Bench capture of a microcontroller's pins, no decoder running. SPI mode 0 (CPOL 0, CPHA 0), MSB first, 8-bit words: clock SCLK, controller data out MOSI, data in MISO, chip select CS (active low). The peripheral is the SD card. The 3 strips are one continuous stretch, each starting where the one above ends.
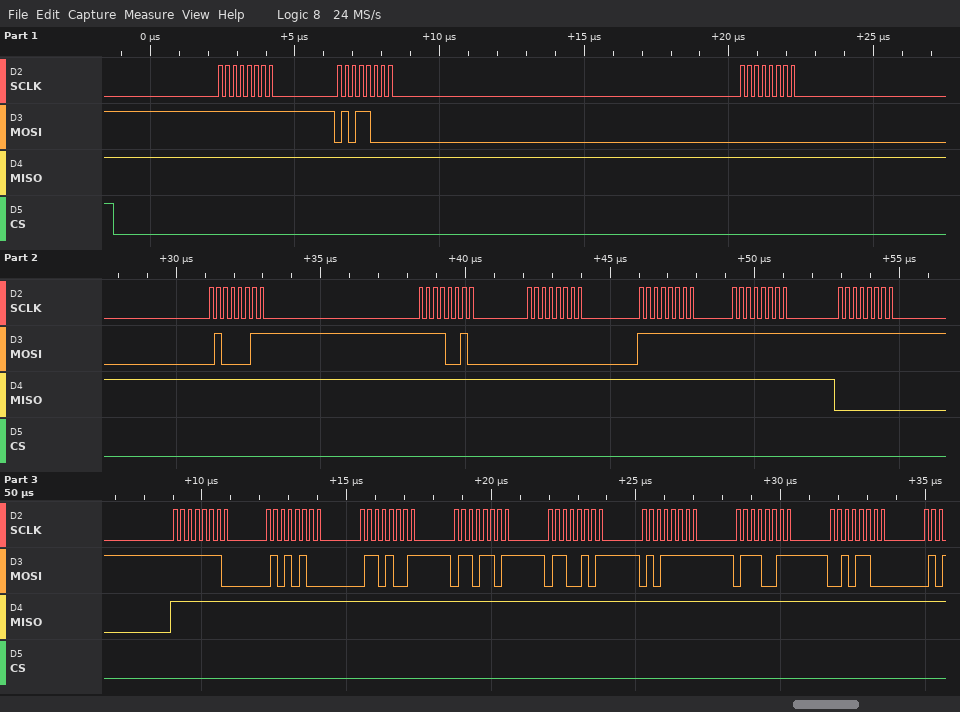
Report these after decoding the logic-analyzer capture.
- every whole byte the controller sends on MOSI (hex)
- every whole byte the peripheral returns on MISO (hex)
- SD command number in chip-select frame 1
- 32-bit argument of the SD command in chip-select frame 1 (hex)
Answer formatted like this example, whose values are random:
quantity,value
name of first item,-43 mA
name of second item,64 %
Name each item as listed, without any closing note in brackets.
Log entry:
quantity,value
every whole byte the controller sends on MOSI,0xFF 0x58 0x00 0x43 0xF2 0x00 0xFF 0xFF 0xFF 0xFE 0x54 0x69 0x6D 0x65 0x5F 0x73 0x2C
every whole byte the peripheral returns on MISO,0xFF 0xFF 0xFF 0xFF 0xFF 0xFF 0xFF 0xFF 0x00 0xFF 0xFF 0xFF 0xFF 0xFF 0xFF 0xFF 0xFF
SD command number in chip-select frame 1,CMD24
32-bit argument of the SD command in chip-select frame 1,0x0043F200
